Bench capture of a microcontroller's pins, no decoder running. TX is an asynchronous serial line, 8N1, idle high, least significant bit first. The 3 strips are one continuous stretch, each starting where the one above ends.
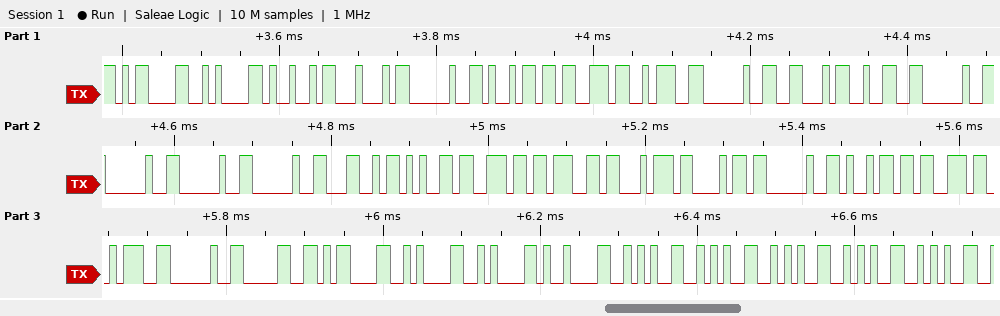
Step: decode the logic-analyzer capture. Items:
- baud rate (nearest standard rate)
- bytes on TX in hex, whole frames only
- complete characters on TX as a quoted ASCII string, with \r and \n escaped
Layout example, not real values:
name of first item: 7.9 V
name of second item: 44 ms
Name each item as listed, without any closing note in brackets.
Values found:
baud rate: 115200 baud
bytes on TX in hex, whole frames only: 0D 0A 49 44 20 69 73 3A 20 46 32 20 20 20 20 4C 65 6E 67 74 68 20 69 73 3A 20 30 0D 0A 0A 09 2A 2A 2A 2A 2A
complete characters on TX as a quoted ASCII string, with \r and \n escaped: "\r\nID is: F2    Length is: 0\r\n\n\t*****"
